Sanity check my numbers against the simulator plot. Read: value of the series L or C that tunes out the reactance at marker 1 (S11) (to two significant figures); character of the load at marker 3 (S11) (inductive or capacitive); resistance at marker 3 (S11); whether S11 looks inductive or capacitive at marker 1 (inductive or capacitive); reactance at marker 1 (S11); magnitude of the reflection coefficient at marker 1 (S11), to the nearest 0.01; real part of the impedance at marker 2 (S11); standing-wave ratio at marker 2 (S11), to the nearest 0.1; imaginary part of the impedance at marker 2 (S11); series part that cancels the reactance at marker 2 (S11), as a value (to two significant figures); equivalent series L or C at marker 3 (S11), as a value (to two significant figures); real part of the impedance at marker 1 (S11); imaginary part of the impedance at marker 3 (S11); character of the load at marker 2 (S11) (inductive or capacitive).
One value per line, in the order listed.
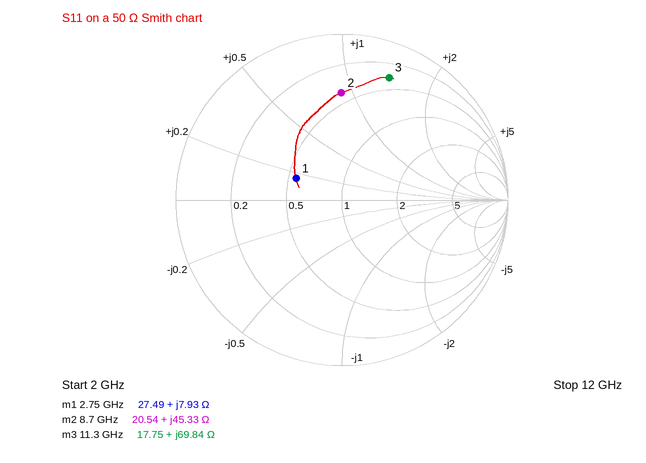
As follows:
7.3 pF
inductive
17.75 Ω
inductive
+7.93 Ω
0.31
20.54 Ω
4.6
+45.33 Ω
400 fF
980 pH
27.49 Ω
+69.84 Ω
inductive
